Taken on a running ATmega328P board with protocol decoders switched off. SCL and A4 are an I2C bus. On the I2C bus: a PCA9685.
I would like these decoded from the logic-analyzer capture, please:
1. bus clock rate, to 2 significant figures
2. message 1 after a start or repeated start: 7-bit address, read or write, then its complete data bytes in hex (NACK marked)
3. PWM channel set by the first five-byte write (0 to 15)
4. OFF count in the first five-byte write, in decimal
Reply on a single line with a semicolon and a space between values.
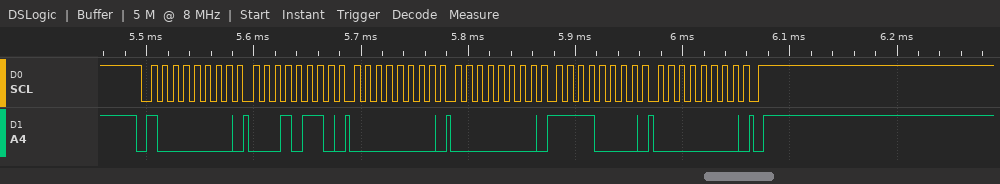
100 kHz; 0x40 write: 16 00 00 F0 00; 4; 240
